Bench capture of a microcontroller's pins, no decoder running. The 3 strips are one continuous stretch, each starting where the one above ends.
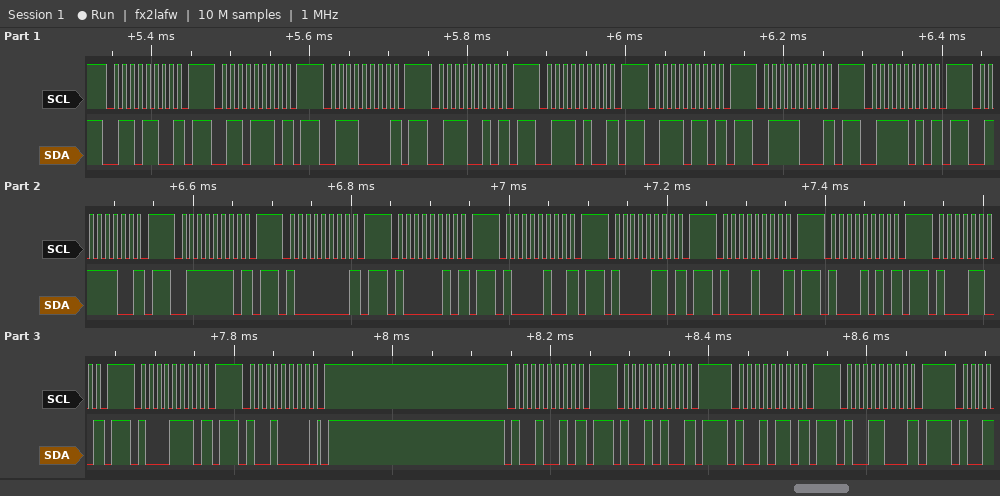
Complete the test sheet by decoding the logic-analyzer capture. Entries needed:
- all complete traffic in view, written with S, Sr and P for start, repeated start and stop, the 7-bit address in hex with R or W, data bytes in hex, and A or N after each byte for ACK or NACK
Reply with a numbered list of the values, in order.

1. S 36W N P S 37W N P S 38W N P S 39W N P S 3AW N P S 3BW N P S 3CW N P S 3DW N P S 3EW N P S 3FW N P S 40W N P S 41W N P S 42W N P S 43W N P S 44W N P S 45W N P S 46W N P S 47W N P S 48W A P S 49W N P S 4AW N P S 4BW N P S 4CW N P
